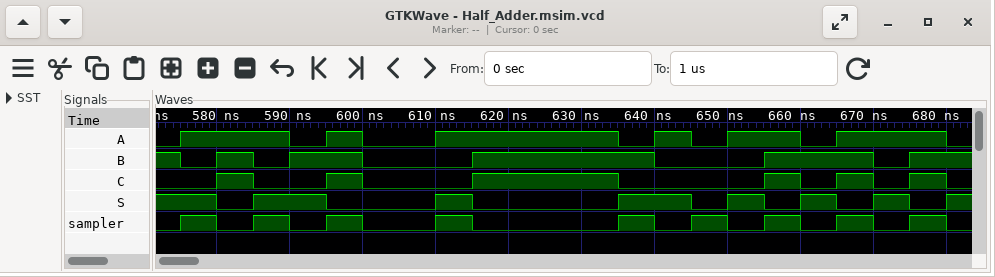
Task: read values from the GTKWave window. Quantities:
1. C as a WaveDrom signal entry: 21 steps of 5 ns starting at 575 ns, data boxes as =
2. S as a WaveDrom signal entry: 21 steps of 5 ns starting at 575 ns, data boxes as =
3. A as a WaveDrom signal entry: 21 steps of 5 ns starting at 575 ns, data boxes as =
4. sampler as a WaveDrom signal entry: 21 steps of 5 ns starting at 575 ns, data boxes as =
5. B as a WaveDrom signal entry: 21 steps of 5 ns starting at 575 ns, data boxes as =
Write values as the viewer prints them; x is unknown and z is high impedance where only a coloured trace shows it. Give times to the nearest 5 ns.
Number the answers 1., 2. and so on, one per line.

1. {name: 'C', wave: '010.10..1...0...10101'}
2. {name: 'S', wave: '101.0..10...1.0101010'}
3. {name: 'A', wave: '1..010.1....0101.01..'}
4. {name: 'sampler', wave: '101010.10...101010101'}
5. {name: 'B', wave: '0101.0..1....0..1..01'}
